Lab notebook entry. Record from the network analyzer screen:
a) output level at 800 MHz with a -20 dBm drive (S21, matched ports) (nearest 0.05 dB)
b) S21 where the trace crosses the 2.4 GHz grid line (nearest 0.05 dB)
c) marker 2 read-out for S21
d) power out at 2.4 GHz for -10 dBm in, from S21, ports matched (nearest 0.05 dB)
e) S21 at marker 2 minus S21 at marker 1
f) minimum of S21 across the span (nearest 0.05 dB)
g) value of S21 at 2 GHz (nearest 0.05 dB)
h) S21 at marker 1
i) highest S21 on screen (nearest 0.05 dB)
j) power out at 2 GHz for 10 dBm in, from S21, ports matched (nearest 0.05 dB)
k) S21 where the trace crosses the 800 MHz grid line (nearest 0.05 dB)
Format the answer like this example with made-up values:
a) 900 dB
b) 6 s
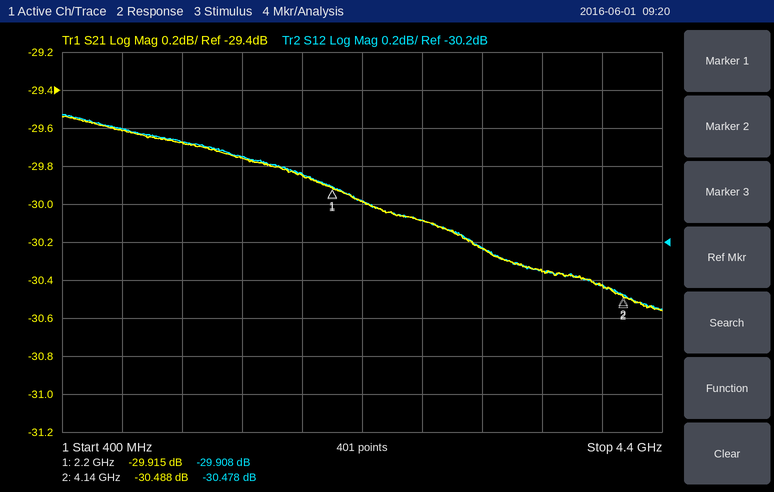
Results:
a) -49.60 dBm
b) -30.00 dB
c) -30.488 dB
d) -40.00 dBm
e) -0.573 dB
f) -30.55 dB
g) -29.85 dB
h) -29.915 dB
i) -29.55 dB
j) -19.85 dBm
k) -29.60 dB
